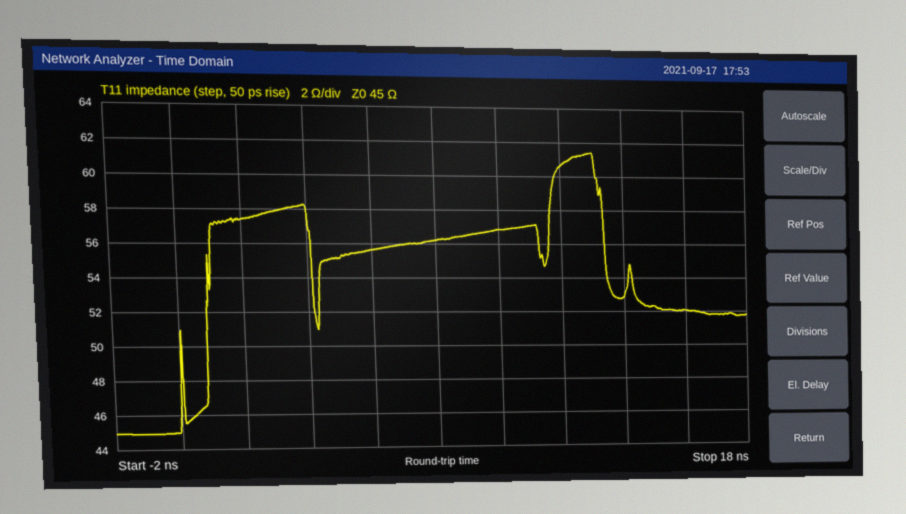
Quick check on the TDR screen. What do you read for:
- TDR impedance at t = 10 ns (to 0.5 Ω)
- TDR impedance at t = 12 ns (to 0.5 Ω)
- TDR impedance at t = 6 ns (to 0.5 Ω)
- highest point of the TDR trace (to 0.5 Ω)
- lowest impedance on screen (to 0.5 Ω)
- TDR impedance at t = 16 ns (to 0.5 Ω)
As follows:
57.0 Ω
60.5 Ω
55.5 Ω
61.5 Ω
45.0 Ω
52.0 Ω
